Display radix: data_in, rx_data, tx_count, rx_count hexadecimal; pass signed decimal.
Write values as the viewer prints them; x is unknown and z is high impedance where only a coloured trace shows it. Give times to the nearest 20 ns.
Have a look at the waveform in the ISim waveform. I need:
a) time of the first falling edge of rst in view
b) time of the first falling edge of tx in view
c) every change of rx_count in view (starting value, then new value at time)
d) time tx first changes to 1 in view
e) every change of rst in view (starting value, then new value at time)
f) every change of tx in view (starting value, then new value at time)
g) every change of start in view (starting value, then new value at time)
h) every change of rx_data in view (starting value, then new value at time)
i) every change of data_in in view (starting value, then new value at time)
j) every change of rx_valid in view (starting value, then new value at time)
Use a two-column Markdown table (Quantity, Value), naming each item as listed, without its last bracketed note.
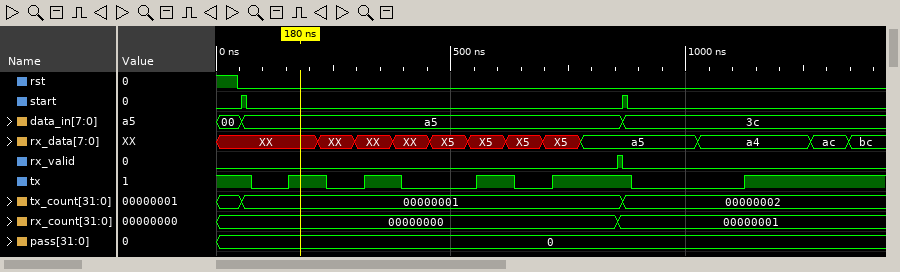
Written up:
| Quantity | Value |
|---|---|
| time of the first falling edge of rst in view | 40 ns |
| time of the first falling edge of tx in view | 80 ns |
| every change of rx_count in view | 00000000, 00000001 at 860 ns |
| time tx first changes to 1 in view | 160 ns |
| every change of rst in view | 1, 0 at 40 ns |
| every change of tx in view | 1, 0 at 80 ns, 1 at 160 ns, 0 at 240 ns, 1 at 320 ns, 0 at 400 ns, 1 at 560 ns, 0 at 640 ns, 1 at 720 ns, 0 at 880 ns, 1 at 1120 ns |
| every change of start in view | 0, 1 at 60 ns, 0 at 60 ns, 1 at 860 ns, 0 at 880 ns |
| every change of rx_data in view | XX, XX at 220 ns, XX at 300 ns, XX at 380 ns, X5 at 460 ns, X5 at 540 ns, X5 at 620 ns, X5 at 700 ns, a5 at 780 ns, a4 at 1020 ns, ac at 1260 ns, bc at 1340 ns |
| every change of data_in in view | 00, a5 at 60 ns, 3c at 860 ns |
| every change of rx_valid in view | 0, 1 at 860 ns, 0 at 860 ns |
